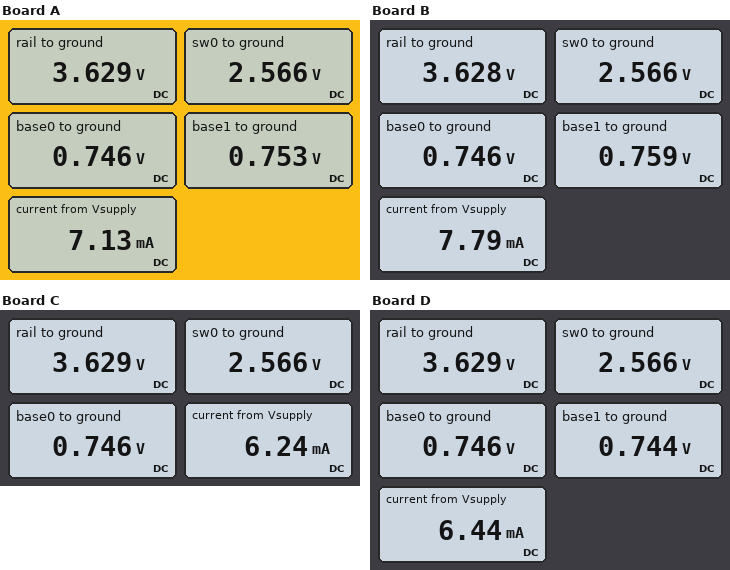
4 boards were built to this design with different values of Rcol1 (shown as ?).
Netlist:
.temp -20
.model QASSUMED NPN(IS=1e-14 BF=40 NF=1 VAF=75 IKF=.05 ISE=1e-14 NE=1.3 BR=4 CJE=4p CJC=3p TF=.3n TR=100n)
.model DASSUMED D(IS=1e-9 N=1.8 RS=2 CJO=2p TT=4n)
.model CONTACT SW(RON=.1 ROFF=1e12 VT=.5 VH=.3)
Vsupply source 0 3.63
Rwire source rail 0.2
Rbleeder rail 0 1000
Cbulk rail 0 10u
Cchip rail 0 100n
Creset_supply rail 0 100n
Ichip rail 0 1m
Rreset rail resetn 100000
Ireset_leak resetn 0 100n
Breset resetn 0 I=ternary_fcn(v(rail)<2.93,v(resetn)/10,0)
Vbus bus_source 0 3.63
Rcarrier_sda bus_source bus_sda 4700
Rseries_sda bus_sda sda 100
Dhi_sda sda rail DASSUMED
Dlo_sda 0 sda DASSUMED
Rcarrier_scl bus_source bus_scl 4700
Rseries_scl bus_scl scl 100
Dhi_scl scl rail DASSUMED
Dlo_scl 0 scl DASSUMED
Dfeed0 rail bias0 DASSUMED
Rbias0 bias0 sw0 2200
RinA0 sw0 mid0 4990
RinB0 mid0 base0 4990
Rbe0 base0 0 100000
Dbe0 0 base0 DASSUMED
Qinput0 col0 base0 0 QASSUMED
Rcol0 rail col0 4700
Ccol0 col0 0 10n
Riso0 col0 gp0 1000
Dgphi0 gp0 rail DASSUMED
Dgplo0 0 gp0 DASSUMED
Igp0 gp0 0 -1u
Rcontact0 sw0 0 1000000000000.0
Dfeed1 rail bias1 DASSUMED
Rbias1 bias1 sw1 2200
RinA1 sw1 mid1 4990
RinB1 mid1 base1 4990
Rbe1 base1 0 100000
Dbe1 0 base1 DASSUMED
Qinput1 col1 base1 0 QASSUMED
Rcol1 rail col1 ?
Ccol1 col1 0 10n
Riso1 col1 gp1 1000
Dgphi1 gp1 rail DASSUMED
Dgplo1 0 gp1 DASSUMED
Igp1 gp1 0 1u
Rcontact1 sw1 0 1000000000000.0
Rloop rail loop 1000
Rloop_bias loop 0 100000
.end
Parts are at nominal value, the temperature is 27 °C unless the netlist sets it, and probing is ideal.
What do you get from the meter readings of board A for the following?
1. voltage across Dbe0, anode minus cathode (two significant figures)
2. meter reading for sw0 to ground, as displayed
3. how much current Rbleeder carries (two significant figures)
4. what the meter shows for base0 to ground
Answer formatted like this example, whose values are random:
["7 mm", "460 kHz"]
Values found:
["-750 mV", "2.566 V", "3.6 mA", "0.746 V"]
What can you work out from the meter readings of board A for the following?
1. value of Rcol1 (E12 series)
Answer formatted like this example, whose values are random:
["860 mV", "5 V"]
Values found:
["2.7 kΩ"]
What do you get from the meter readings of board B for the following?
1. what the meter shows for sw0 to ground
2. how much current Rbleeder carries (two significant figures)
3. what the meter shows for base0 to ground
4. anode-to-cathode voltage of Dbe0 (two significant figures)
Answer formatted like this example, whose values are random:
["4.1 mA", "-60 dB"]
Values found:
["2.566 V", "3.6 mA", "0.746 V", "-750 mV"]
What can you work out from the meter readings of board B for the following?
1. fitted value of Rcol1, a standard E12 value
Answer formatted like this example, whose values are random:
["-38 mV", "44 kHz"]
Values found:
["1.8 kΩ"]
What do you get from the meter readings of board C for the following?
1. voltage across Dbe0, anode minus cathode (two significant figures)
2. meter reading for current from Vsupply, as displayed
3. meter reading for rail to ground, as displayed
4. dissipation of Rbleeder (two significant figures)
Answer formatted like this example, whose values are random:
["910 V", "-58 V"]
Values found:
["-750 mV", "6.24 mA", "3.629 V", "13 mW"]
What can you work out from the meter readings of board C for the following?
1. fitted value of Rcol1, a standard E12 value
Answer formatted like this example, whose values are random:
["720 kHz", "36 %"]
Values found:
["8.2 kΩ"]
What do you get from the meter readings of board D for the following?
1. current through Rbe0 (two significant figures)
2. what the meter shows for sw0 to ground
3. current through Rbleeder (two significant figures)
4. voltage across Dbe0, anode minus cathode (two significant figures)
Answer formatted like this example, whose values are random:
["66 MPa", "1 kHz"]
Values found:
["7.5 µA", "2.566 V", "3.6 mA", "-750 mV"]
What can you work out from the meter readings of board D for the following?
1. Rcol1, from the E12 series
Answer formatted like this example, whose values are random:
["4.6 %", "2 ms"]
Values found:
["5.6 kΩ"]
